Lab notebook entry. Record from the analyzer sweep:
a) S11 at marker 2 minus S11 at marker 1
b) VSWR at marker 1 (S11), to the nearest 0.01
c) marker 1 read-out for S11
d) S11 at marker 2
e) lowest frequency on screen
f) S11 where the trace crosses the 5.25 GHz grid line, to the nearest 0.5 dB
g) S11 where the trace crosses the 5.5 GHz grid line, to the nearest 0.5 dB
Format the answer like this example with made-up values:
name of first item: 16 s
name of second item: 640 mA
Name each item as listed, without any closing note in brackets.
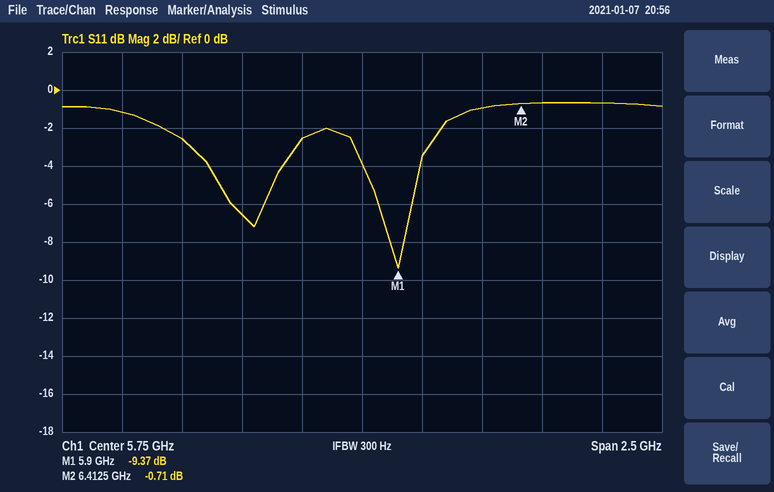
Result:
S11 at marker 2 minus S11 at marker 1: 8.66 dB
VSWR at marker 1 (S11), to the nearest 0.01: 2.03
marker 1 read-out for S11: -9.37 dB
S11 at marker 2: -0.71 dB
lowest frequency on screen: 4.5 GHz
S11 where the trace crosses the 5.25 GHz grid line, to the nearest 0.5 dB: -6.5 dB
S11 where the trace crosses the 5.5 GHz grid line, to the nearest 0.5 dB: -2.5 dB
